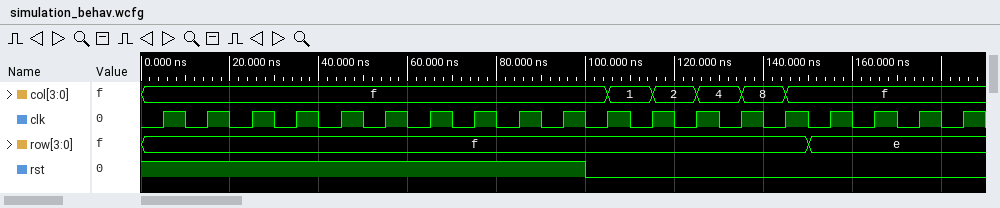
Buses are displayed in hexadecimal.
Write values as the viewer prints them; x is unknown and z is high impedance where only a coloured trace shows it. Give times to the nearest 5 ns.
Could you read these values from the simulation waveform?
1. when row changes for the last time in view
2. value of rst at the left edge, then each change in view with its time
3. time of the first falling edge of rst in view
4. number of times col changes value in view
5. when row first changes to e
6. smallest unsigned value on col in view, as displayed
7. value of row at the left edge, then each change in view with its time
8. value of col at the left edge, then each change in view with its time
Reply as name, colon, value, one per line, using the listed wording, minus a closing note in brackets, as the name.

when row changes for the last time in view: 150 ns
value of rst at the left edge, then each change in view with its time: 1, 0 at 100 ns
time of the first falling edge of rst in view: 100 ns
number of times col changes value in view: 5
when row first changes to e: 150 ns
smallest unsigned value on col in view, as displayed: 1
value of row at the left edge, then each change in view with its time: f, e at 150 ns
value of col at the left edge, then each change in view with its time: f, 1 at 105 ns, 2 at 115 ns, 4 at 125 ns, 8 at 135 ns, f at 145 ns
